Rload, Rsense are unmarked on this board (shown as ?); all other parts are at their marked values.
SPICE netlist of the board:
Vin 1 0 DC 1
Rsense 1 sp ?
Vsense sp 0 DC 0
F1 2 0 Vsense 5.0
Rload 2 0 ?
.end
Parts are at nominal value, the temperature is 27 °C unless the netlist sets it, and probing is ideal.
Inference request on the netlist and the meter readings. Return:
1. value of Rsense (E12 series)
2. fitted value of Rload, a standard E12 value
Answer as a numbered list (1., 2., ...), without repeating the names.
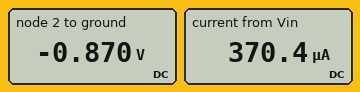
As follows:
1. 2.7 kΩ
2. 470 Ω
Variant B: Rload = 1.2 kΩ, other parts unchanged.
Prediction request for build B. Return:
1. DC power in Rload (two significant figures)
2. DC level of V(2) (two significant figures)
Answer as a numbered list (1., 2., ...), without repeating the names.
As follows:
1. 4.1 mW
2. -2.2 V
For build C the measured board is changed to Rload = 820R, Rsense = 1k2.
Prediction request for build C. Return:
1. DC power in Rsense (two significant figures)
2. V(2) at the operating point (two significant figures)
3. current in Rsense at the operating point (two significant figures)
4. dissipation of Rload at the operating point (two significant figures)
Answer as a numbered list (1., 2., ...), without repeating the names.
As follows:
1. 830 µW
2. -3.4 V
3. 830 µA
4. 14 mW
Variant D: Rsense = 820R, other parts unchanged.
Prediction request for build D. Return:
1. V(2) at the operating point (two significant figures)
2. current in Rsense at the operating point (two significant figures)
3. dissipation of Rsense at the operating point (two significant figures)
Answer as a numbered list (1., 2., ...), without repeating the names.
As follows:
1. -2.9 V
2. 1.2 mA
3. 1.2 mW
